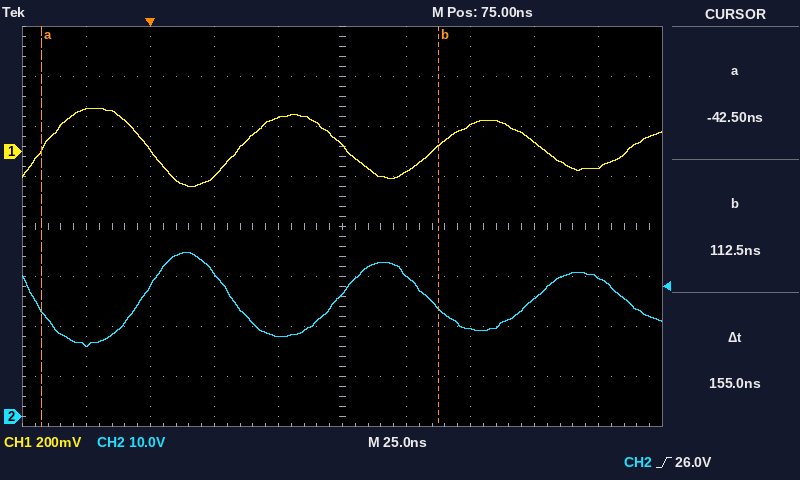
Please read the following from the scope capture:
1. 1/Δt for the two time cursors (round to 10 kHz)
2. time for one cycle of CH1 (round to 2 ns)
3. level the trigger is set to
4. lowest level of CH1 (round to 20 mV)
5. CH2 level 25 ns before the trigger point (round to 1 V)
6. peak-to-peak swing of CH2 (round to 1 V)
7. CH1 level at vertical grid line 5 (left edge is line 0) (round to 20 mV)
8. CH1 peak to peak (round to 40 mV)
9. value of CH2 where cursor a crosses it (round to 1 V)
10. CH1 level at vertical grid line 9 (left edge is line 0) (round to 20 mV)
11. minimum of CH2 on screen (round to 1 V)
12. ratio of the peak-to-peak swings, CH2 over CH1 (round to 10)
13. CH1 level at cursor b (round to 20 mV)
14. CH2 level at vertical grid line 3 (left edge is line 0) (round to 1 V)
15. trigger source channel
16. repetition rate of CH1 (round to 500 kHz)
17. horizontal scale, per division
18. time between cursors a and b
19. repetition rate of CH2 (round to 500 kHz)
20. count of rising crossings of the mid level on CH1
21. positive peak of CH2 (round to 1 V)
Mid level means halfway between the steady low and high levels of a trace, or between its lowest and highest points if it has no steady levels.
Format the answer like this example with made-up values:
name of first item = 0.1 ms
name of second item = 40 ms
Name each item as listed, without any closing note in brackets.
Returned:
1/Δt for the two time cursors = 6.45 MHz
time for one cycle of CH1 = 76 ns
level the trigger is set to = 26.0 V
lowest level of CH1 = -140 mV
CH2 level 25 ns before the trigger point = 14 V
peak-to-peak swing of CH2 = 19 V
CH1 level at vertical grid line 5 (left edge is line 0) = 20 mV
CH1 peak to peak = 320 mV
value of CH2 where cursor a crosses it = 21 V
CH1 level at vertical grid line 9 (left edge is line 0) = -60 mV
minimum of CH2 on screen = 14 V
ratio of the peak-to-peak swings, CH2 over CH1 = 60
CH1 level at cursor b = 20 mV
CH2 level at vertical grid line 3 (left edge is line 0) = 29 V
trigger source channel = CH2
repetition rate of CH1 = 13.0 MHz
horizontal scale, per division = 25 ns
time between cursors a and b = 155 ns
repetition rate of CH2 = 13.0 MHz
count of rising crossings of the mid level on CH1 = 4
positive peak of CH2 = 33 V
